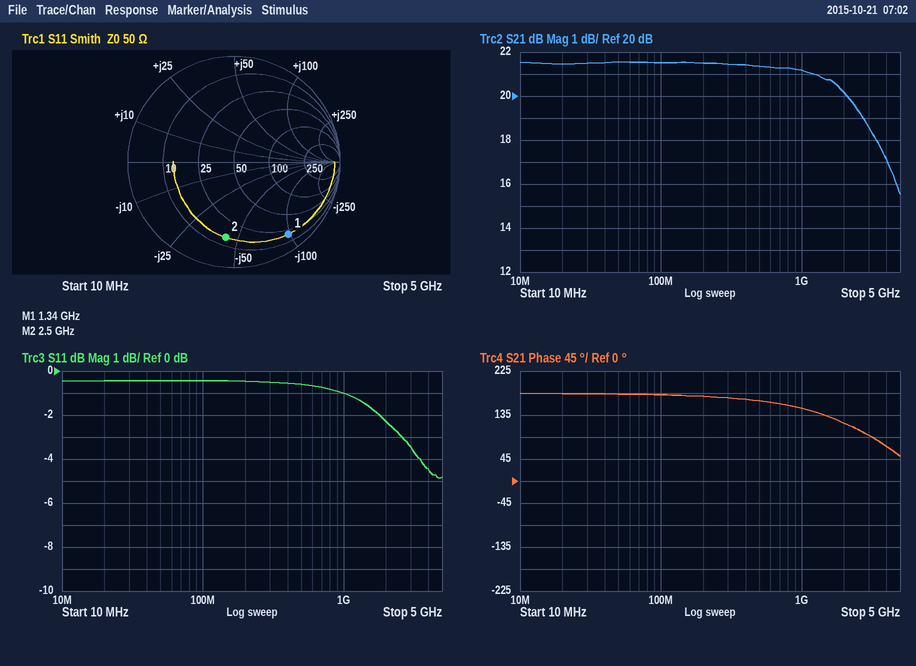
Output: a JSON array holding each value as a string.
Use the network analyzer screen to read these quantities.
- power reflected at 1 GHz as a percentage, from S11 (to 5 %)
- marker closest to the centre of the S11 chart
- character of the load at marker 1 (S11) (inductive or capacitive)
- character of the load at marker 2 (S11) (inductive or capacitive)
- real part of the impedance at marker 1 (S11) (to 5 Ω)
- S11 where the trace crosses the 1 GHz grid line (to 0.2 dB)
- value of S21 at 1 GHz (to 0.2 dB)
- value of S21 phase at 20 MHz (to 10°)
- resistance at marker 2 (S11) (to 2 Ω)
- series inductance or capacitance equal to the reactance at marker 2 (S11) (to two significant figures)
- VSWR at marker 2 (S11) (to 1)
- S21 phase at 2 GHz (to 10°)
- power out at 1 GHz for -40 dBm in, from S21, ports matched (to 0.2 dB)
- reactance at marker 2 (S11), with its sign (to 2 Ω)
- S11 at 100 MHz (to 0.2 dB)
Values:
["80 %", "marker 2", "capacitive", "capacitive", "20 Ω", "-1.0 dB", "21.2 dB", "180°", "14 Ω", "1.5 pF", "6", "120°", "-18.8 dBm", "-42 Ω", "-0.4 dB"]
